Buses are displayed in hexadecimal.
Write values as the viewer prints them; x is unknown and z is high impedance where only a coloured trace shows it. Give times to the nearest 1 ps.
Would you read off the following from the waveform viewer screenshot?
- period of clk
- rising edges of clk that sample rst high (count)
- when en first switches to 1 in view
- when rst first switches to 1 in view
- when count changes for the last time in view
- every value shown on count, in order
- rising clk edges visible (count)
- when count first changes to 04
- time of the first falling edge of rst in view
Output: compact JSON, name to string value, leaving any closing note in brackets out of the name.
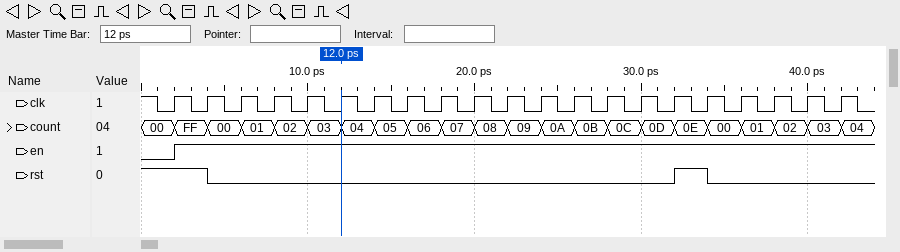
{"period of clk": "2 ps", "rising edges of clk that sample rst high": "3", "when en first switches to 1 in view": "2 ps", "when rst first switches to 1 in view": "32 ps", "when count changes for the last time in view": "42 ps", "every value shown on count, in order": "00, FF, 00, 01, 02, 03, 04, 05, 06, 07, 08, 09, 0A, 0B, 0C, 0D, 0E, 00, 01, 02, 03, 04", "rising clk edges visible": "21", "when count first changes to 04": "12 ps", "time of the first falling edge of rst in view": "4 ps"}
